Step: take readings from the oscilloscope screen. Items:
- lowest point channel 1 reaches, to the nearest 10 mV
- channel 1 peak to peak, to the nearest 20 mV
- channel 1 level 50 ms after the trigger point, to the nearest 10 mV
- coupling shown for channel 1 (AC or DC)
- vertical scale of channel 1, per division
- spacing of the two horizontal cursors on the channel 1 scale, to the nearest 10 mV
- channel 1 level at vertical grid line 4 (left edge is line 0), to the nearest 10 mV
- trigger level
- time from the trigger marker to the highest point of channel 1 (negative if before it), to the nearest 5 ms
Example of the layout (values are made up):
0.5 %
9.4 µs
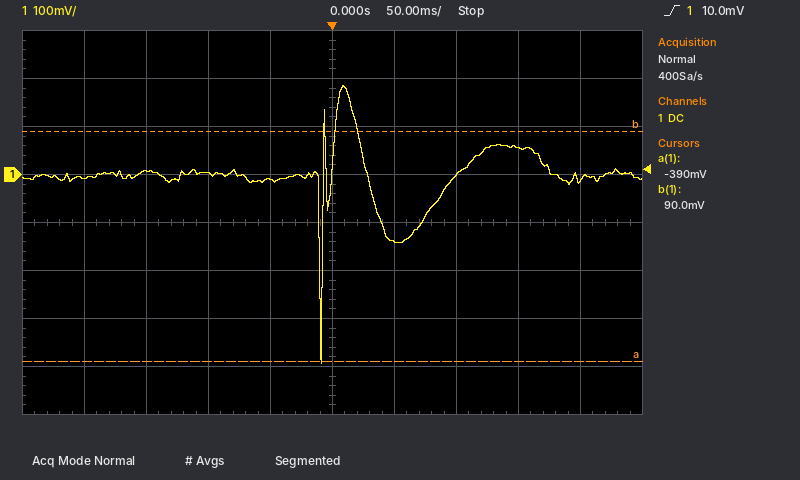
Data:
-390 mV
580 mV
-140 mV
DC
100 mV
480 mV
-10 mV
10.0 mV
+10 ms
